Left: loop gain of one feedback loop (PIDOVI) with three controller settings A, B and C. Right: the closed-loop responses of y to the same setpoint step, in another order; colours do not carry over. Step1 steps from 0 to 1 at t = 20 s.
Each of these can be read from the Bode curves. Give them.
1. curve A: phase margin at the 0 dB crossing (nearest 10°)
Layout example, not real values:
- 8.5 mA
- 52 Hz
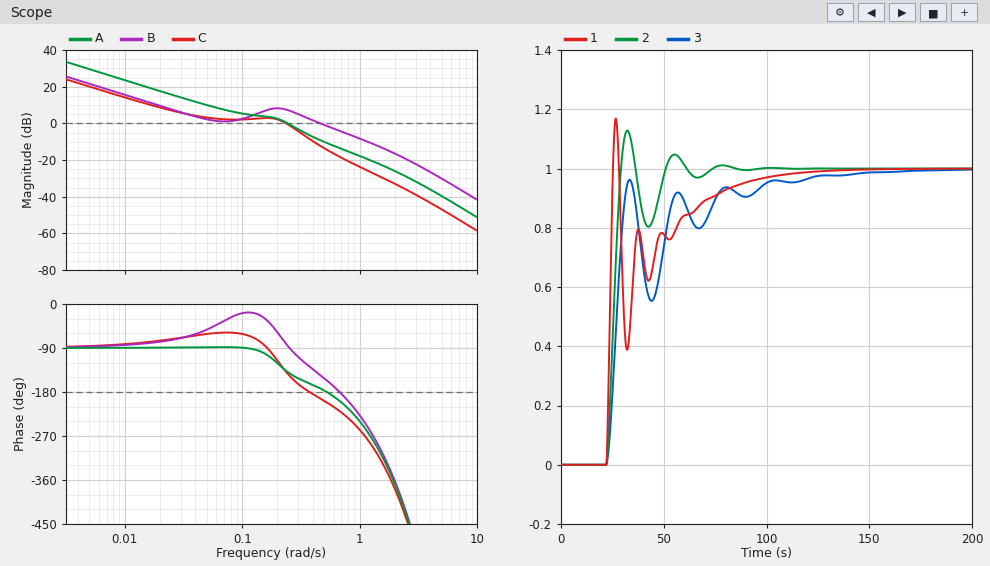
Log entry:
- 40°
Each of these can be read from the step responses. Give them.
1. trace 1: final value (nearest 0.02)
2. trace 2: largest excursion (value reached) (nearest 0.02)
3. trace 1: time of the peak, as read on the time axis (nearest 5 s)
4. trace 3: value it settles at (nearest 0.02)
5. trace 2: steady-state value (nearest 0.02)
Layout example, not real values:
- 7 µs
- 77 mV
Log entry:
- 1.00
- 1.12
- 25 s
- 1.00
- 1.00
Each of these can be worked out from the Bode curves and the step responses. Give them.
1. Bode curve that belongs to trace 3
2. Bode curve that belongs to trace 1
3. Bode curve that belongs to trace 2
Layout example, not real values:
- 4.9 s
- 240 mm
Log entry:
- C
- B
- A
